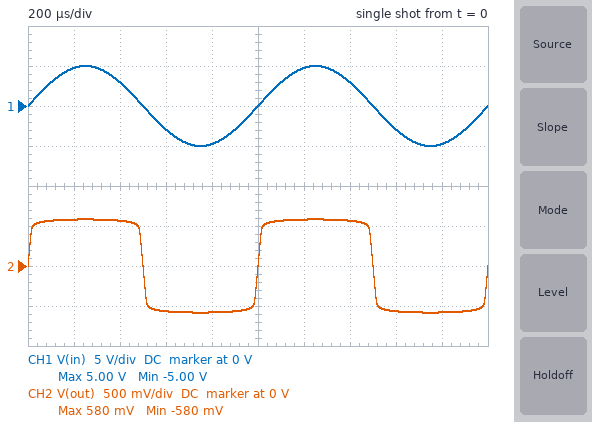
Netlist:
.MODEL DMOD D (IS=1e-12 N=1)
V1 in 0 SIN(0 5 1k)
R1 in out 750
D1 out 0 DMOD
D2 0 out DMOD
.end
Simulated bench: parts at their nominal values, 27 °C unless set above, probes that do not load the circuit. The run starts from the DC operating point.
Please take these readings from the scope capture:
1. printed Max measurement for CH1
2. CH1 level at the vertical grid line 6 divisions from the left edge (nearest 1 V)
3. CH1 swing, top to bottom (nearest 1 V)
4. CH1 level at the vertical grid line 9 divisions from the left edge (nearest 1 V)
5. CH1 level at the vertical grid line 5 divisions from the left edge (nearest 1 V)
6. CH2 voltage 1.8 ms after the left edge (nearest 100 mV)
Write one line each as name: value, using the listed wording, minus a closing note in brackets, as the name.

printed Max measurement for CH1: 5.00 V
CH1 level at the vertical grid line 6 divisions from the left edge: 5 V
CH1 swing, top to bottom: 10 V
CH1 level at the vertical grid line 9 divisions from the left edge: -5 V
CH1 level at the vertical grid line 5 divisions from the left edge: 0 V
CH2 voltage 1.8 ms after the left edge: -600 mV
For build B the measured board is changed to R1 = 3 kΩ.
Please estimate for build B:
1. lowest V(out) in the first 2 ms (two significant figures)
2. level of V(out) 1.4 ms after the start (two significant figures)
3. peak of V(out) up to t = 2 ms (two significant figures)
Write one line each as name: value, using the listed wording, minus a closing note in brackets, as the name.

lowest V(out) in the first 2 ms: -550 mV
level of V(out) 1.4 ms after the start: 530 mV
peak of V(out) up to t = 2 ms: 550 mV
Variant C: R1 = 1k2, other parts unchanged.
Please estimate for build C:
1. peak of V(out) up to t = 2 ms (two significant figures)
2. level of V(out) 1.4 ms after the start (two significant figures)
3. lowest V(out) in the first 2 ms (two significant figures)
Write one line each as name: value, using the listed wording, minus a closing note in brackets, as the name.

peak of V(out) up to t = 2 ms: 570 mV
level of V(out) 1.4 ms after the start: 550 mV
lowest V(out) in the first 2 ms: -570 mV
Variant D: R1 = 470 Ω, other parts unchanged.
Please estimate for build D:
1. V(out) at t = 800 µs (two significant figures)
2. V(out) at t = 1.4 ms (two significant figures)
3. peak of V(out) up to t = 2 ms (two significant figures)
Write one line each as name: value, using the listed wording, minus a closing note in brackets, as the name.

V(out) at t = 800 µs: -590 mV
V(out) at t = 1.4 ms: 580 mV
peak of V(out) up to t = 2 ms: 590 mV
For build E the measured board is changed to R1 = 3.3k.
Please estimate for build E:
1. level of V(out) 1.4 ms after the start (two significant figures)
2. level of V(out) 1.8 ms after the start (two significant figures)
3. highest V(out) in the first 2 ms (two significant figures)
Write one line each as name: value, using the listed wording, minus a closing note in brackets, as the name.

level of V(out) 1.4 ms after the start: 530 mV
level of V(out) 1.8 ms after the start: -540 mV
highest V(out) in the first 2 ms: 540 mV
